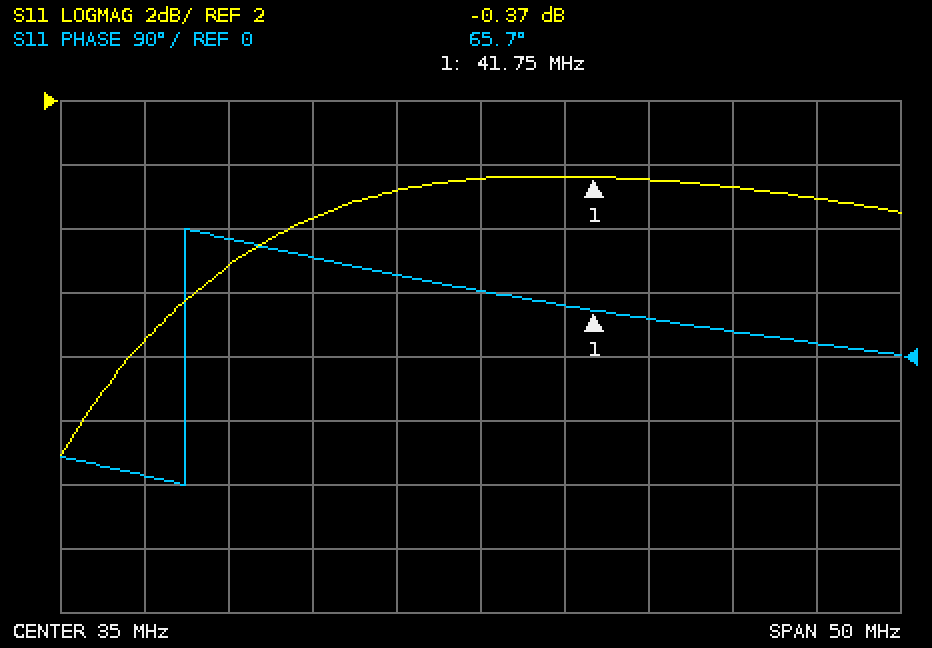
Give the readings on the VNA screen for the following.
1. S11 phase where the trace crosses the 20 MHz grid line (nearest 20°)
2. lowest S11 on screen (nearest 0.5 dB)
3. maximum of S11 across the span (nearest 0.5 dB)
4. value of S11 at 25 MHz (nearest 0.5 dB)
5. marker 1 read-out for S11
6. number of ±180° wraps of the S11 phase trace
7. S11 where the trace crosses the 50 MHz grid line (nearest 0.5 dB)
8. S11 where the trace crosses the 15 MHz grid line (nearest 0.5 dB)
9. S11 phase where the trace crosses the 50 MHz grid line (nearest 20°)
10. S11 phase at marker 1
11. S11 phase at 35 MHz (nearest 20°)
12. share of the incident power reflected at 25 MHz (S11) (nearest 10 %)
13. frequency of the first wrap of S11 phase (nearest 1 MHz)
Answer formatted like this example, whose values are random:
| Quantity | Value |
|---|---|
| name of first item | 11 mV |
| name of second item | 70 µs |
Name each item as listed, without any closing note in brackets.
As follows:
| Quantity | Value |
|---|---|
| S11 phase where the trace crosses the 20 MHz grid line | 160° |
| lowest S11 on screen | -9.0 dB |
| maximum of S11 across the span | -0.5 dB |
| value of S11 at 25 MHz | -1.5 dB |
| marker 1 read-out for S11 | -0.37 dB |
| number of ±180° wraps of the S11 phase trace | 1 |
| S11 where the trace crosses the 50 MHz grid line | -0.5 dB |
| S11 where the trace crosses the 15 MHz grid line | -5.5 dB |
| S11 phase where the trace crosses the 50 MHz grid line | 40° |
| S11 phase at marker 1 | 65.7° |
| S11 phase at 35 MHz | 100° |
| share of the incident power reflected at 25 MHz (S11) | 70 % |
| frequency of the first wrap of S11 phase | 17 MHz |
